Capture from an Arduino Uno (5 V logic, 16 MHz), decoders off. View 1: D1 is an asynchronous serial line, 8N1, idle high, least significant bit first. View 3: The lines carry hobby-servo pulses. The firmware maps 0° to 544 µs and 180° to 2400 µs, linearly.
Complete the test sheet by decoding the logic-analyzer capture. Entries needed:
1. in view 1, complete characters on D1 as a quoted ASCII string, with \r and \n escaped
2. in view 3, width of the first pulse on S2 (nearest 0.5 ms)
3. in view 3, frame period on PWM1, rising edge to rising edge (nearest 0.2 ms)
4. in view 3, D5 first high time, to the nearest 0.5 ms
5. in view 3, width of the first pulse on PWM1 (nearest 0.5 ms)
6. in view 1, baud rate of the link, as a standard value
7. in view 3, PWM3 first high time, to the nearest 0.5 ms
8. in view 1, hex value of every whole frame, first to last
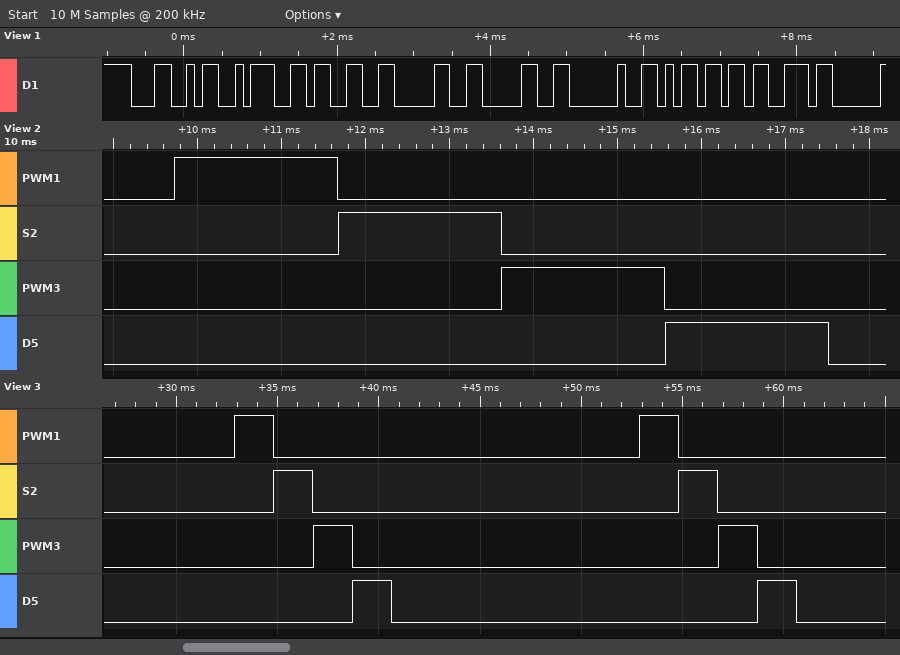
"L:300 ms"
2.0 ms
20.0 ms
2.0 ms
2.0 ms
9600 baud
2.0 ms
4C 3A 33 30 30 20 6D 73
